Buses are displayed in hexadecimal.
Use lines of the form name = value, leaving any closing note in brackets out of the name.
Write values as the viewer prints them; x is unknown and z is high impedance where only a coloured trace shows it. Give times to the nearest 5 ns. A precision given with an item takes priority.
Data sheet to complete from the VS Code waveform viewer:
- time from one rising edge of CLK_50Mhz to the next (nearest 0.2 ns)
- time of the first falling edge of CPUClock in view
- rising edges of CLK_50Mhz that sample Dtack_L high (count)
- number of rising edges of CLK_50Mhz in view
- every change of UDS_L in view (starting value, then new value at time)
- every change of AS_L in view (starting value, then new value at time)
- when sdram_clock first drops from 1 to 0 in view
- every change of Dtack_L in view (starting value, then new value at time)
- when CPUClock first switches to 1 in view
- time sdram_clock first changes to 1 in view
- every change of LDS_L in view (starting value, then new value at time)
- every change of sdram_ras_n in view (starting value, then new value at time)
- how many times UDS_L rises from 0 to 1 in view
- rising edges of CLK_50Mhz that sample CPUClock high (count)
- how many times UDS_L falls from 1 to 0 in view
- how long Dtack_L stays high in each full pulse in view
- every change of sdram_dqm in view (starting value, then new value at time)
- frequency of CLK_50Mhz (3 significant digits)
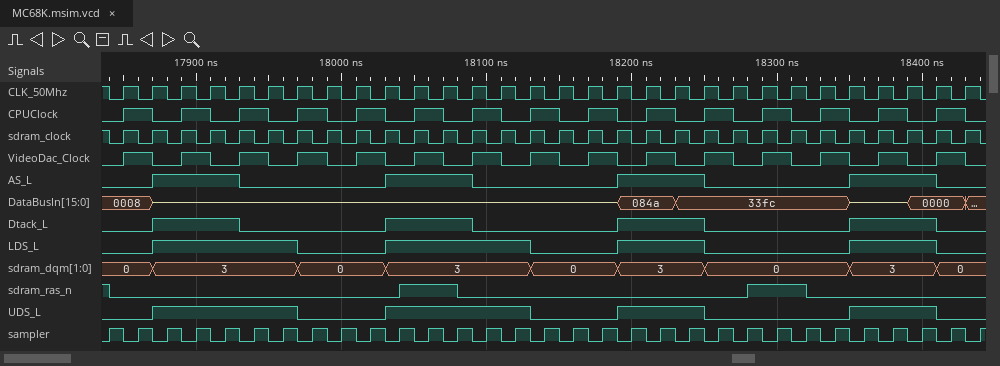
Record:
time from one rising edge of CLK_50Mhz to the next = 20 ns
time of the first falling edge of CPUClock in view = 17870 ns
rising edges of CLK_50Mhz that sample Dtack_L high = 12
number of rising edges of CLK_50Mhz in view = 30
every change of UDS_L in view = 0, 1 at 17870 ns, 0 at 17970 ns, 1 at 18030 ns, 0 at 18130 ns, 1 at 18190 ns, 0 at 18250 ns, 1 at 18350 ns, 0 at 18410 ns
every change of AS_L in view = 0, 1 at 17870 ns, 0 at 17930 ns, 1 at 18030 ns, 0 at 18090 ns, 1 at 18190 ns, 0 at 18250 ns, 1 at 18350 ns, 0 at 18410 ns
when sdram_clock first drops from 1 to 0 in view = 17840 ns
every change of Dtack_L in view = 0, 1 at 17870 ns, 0 at 17930 ns, 1 at 18030 ns, 0 at 18090 ns, 1 at 18190 ns, 0 at 18250 ns, 1 at 18350 ns, 0 at 18410 ns
when CPUClock first switches to 1 in view = 17850 ns
time sdram_clock first changes to 1 in view = 17850 ns
every change of LDS_L in view = 0, 1 at 17870 ns, 0 at 17970 ns, 1 at 18030 ns, 0 at 18130 ns, 1 at 18190 ns, 0 at 18250 ns, 1 at 18350 ns, 0 at 18410 ns
every change of sdram_ras_n in view = 1, 0 at 17840 ns, 1 at 18040 ns, 0 at 18080 ns, 1 at 18280 ns, 0 at 18320 ns
how many times UDS_L rises from 0 to 1 in view = 4
rising edges of CLK_50Mhz that sample CPUClock high = 15
how many times UDS_L falls from 1 to 0 in view = 4
how long Dtack_L stays high in each full pulse in view = 60 ns, 60 ns, 60 ns, 60 ns
every change of sdram_dqm in view = 0, 3 at 17870 ns, 0 at 17970 ns, 3 at 18030 ns, 0 at 18130 ns, 3 at 18190 ns, 0 at 18250 ns, 3 at 18350 ns, 0 at 18410 ns
frequency of CLK_50Mhz = 50.0 MHz
